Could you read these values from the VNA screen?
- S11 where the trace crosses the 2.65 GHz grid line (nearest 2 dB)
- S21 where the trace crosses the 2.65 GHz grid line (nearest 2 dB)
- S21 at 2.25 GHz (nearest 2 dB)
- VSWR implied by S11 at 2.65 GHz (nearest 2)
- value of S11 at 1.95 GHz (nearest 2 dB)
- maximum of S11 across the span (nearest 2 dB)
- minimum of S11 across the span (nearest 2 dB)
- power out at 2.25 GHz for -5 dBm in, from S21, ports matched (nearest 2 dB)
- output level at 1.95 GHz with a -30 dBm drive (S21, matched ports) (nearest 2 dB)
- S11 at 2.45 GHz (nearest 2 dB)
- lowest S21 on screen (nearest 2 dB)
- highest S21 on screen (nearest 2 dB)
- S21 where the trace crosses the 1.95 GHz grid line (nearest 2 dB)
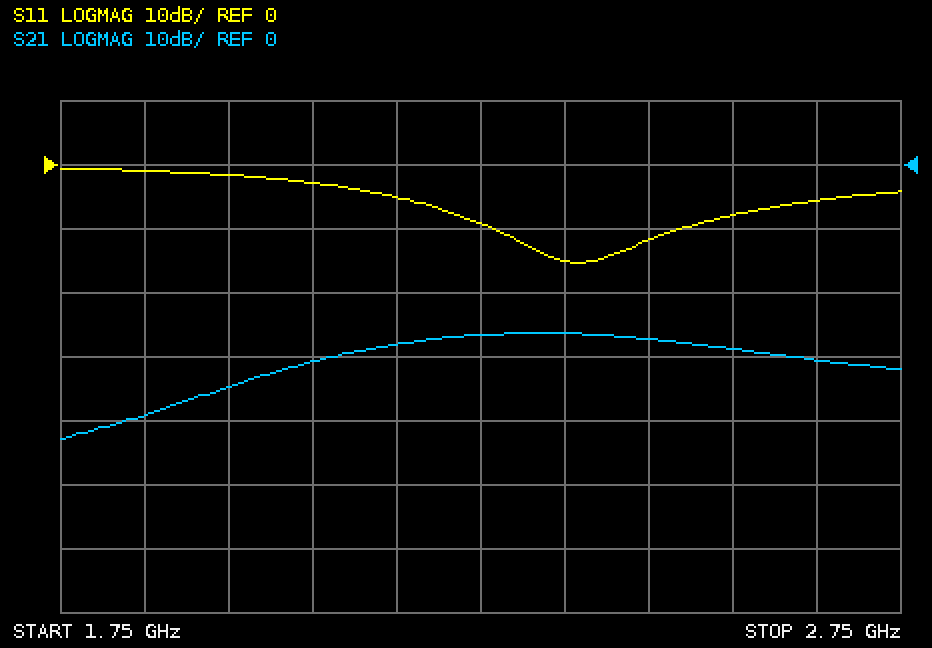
-6 dB
-30 dB
-26 dB
4
-2 dB
0 dB
-16 dB
-32 dBm
-64 dBm
-12 dB
-42 dB
-26 dB
-34 dB
